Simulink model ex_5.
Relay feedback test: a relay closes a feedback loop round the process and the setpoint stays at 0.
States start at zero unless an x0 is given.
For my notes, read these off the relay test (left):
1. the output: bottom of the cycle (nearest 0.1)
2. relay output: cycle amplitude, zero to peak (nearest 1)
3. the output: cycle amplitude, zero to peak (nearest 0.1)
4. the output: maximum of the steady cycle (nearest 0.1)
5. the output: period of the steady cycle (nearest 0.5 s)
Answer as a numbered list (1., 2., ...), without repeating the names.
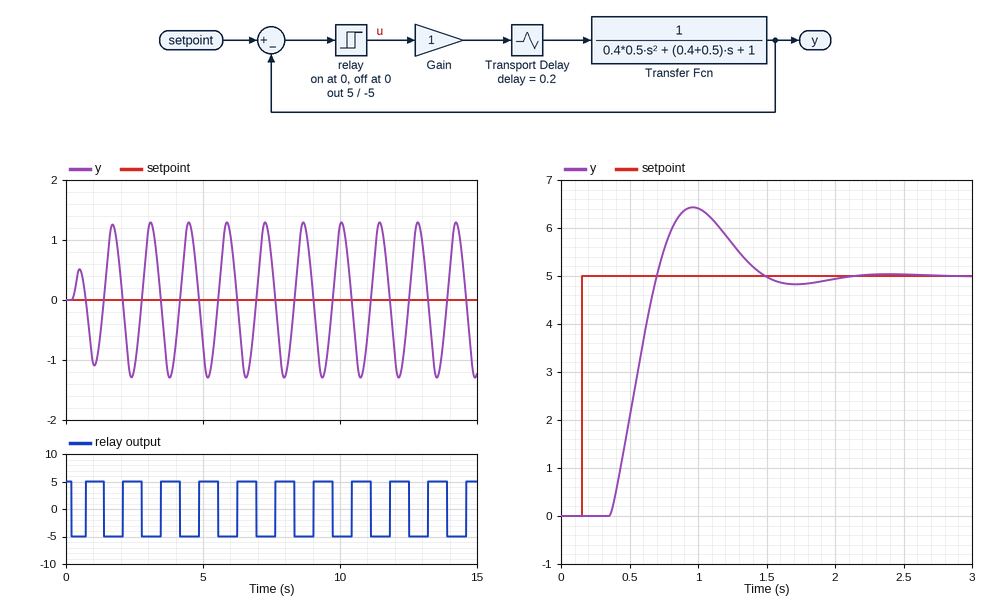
1. -1.3
2. 5
3. 1.3
4. 1.3
5. 1.5 s
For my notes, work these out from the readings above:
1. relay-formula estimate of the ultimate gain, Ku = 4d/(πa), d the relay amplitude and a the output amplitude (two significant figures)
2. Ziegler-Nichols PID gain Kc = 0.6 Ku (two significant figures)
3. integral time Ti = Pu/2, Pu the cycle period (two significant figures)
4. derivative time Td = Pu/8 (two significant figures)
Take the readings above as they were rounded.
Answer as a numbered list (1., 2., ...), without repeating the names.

1. 4.9
2. 2.9
3. 0.75 s
4. 0.19 s
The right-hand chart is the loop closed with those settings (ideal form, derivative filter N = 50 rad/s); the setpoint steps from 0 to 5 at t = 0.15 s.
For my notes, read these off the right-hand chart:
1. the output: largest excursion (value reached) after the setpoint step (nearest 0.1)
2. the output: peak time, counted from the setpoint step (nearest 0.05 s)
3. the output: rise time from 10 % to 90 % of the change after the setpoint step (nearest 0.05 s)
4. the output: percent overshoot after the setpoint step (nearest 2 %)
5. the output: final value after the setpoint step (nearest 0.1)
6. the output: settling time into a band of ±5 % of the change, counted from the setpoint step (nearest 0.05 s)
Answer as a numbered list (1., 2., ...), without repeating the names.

1. 6.4
2. 0.80 s
3. 0.25 s
4. 28 %
5. 5.0
6. 1.25 s
